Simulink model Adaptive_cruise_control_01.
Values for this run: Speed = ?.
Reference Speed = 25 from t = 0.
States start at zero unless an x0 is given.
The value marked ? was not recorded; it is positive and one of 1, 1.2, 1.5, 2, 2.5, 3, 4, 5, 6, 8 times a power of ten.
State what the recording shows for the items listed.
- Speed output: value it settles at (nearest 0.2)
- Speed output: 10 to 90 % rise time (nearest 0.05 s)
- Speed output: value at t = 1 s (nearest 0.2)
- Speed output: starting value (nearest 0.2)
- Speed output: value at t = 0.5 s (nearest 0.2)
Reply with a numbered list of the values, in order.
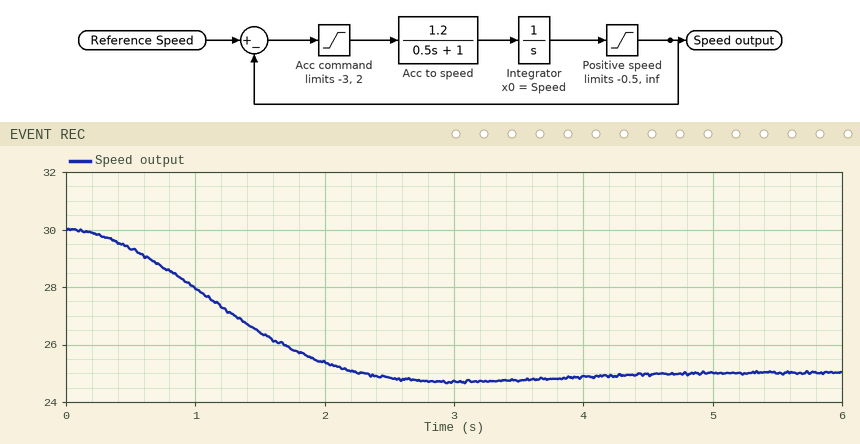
1. 25.0
2. 1.50 s
3. 28.0
4. 30.0
5. 29.4
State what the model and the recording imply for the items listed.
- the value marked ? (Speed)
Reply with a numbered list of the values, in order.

1. 30
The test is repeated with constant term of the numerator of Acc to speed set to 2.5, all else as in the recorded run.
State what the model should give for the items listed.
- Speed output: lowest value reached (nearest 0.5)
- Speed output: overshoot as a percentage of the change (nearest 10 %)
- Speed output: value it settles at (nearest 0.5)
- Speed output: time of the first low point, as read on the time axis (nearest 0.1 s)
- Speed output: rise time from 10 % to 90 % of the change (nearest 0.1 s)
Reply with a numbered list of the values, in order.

1. 24.0
2. 20 %
3. 25.0
4. 1.8 s
5. 0.8 s
